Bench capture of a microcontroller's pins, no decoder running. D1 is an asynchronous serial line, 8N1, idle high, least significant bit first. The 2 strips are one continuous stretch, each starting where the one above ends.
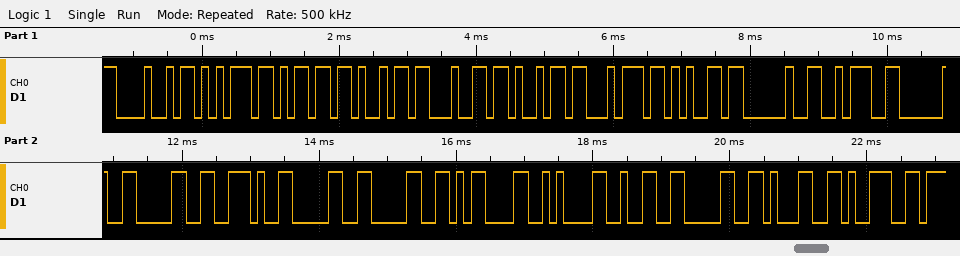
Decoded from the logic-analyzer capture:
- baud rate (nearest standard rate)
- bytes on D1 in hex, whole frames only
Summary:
9600 baud
0x48 0x75 0x6D 0x69 0x64 0x69 0x74 0x65 0x20 0x3A 0x20 0x30 0x2E 0x30 0x30 0x0D 0x0A 0x32 0x30 0x31 0x39
